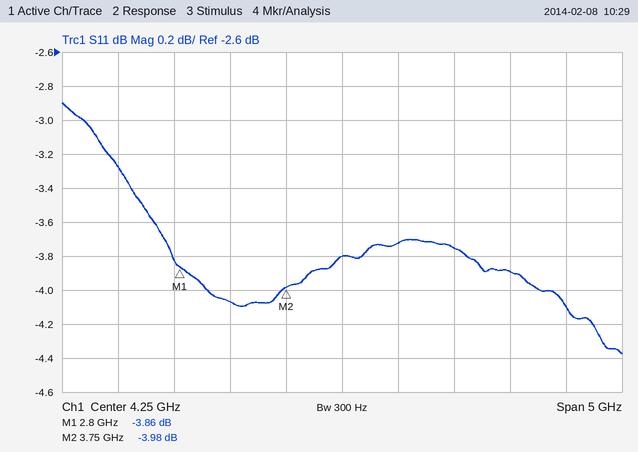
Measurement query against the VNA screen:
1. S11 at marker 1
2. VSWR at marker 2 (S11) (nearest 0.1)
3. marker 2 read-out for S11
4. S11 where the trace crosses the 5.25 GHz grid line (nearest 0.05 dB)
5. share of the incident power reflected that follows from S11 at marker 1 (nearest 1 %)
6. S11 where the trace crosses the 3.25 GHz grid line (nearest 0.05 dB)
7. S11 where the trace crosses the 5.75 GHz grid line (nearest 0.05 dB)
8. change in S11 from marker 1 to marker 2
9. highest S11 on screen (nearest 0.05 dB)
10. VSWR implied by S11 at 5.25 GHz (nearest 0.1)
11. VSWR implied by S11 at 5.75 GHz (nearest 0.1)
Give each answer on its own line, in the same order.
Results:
-3.86 dB
4.4
-3.98 dB
-3.75 dB
41 %
-4.05 dB
-3.90 dB
-0.12 dB
-2.90 dB
4.7
4.5
